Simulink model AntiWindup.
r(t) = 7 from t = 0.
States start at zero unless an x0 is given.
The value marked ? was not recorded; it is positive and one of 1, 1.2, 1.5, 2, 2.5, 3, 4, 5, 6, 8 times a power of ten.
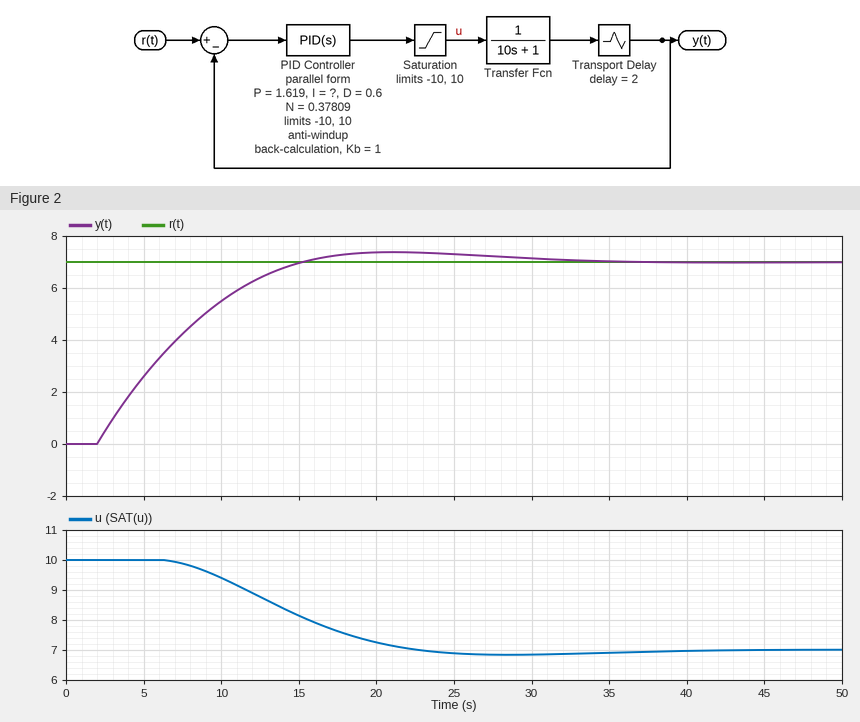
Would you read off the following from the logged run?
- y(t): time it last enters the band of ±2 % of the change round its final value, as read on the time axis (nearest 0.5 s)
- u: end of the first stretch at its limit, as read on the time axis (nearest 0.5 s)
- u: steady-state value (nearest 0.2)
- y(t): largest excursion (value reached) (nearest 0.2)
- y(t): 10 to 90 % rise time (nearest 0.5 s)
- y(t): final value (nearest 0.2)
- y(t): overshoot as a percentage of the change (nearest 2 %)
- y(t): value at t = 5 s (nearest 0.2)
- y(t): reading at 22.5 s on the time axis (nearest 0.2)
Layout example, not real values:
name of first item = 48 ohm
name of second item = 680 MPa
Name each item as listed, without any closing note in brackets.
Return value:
y(t): time it last enters the band of ±2 % of the change round its final value, as read on the time axis = 30.0 s
u: end of the first stretch at its limit, as read on the time axis = 7.0 s
u: steady-state value = 7.0
y(t): largest excursion (value reached) = 7.4
y(t): 10 to 90 % rise time = 9.5 s
y(t): final value = 7.0
y(t): overshoot as a percentage of the change = 6 %
y(t): value at t = 5 s = 2.6
y(t): reading at 22.5 s on the time axis = 7.4
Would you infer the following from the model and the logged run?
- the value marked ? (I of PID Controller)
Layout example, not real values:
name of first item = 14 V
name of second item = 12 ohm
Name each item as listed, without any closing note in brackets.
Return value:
the value marked ? = 0.3
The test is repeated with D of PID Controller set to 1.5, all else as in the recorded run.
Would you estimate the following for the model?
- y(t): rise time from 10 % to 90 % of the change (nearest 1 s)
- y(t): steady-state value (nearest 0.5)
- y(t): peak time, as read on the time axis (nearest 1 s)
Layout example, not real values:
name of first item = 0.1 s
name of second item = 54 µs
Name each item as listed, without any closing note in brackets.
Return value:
y(t): rise time from 10 % to 90 % of the change = 10 s
y(t): steady-state value = 7.0
y(t): peak time, as read on the time axis = 23 s
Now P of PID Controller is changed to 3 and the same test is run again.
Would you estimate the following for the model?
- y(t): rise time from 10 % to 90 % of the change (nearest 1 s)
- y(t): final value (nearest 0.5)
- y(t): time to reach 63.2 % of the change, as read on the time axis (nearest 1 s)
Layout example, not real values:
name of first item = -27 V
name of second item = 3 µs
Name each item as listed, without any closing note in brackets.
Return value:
y(t): rise time from 10 % to 90 % of the change = 20 s
y(t): final value = 7.0
y(t): time to reach 63.2 % of the change, as read on the time axis = 9 s
